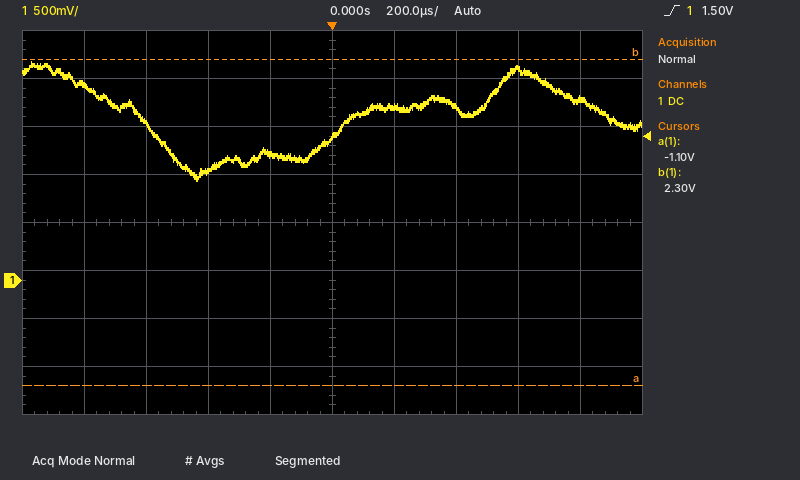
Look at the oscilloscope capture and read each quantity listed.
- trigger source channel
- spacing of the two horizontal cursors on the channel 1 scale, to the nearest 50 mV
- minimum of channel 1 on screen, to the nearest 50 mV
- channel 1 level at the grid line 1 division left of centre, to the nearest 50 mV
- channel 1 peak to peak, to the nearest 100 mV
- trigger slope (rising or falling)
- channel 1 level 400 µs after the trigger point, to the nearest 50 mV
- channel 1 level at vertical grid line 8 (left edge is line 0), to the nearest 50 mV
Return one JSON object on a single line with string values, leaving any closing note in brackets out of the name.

{"trigger source channel": "channel 1", "spacing of the two horizontal cursors on the channel 1 scale, to the nearest 50 mV": "3.40 V", "minimum of channel 1 on screen, to the nearest 50 mV": "1.05 V", "channel 1 level at the grid line 1 division left of centre, to the nearest 50 mV": "1.30 V", "channel 1 peak to peak, to the nearest 100 mV": "1.20 V", "trigger slope": "rising", "channel 1 level 400 µs after the trigger point, to the nearest 50 mV": "1.80 V", "channel 1 level at vertical grid line 8 (left edge is line 0), to the nearest 50 mV": "2.20 V"}
